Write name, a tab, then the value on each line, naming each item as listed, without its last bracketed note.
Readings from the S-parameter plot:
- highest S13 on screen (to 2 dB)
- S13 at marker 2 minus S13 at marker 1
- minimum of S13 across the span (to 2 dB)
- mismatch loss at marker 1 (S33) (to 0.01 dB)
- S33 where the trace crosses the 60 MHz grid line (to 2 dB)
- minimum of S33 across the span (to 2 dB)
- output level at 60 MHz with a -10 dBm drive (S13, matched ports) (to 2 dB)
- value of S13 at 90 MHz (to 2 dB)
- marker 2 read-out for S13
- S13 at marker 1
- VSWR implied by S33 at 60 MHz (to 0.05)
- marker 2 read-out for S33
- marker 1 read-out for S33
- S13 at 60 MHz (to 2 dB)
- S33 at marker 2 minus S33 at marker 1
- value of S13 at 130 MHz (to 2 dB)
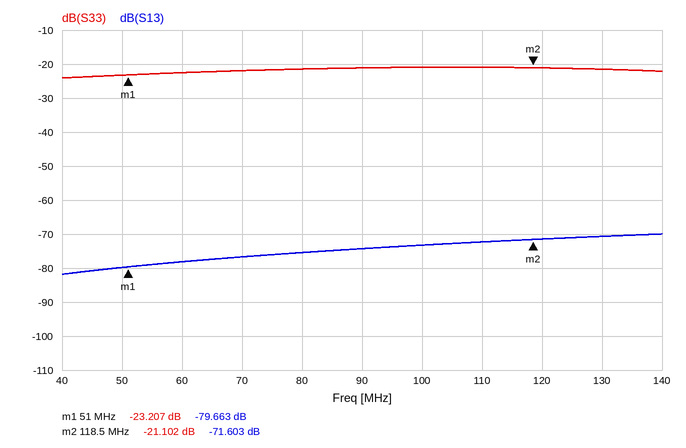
highest S13 on screen	-70 dB
S13 at marker 2 minus S13 at marker 1	8.060 dB
minimum of S13 across the span	-82 dB
mismatch loss at marker 1 (S33)	0.02 dB
S33 where the trace crosses the 60 MHz grid line	-22 dB
minimum of S33 across the span	-24 dB
output level at 60 MHz with a -10 dBm drive (S13, matched ports)	-88 dBm
value of S13 at 90 MHz	-74 dB
marker 2 read-out for S13	-71.603 dB
S13 at marker 1	-79.663 dB
VSWR implied by S33 at 60 MHz	1.15
marker 2 read-out for S33	-21.102 dB
marker 1 read-out for S33	-23.207 dB
S13 at 60 MHz	-78 dB
S33 at marker 2 minus S33 at marker 1	2.105 dB
value of S13 at 130 MHz	-70 dB
